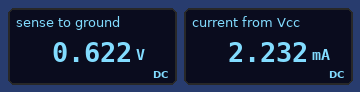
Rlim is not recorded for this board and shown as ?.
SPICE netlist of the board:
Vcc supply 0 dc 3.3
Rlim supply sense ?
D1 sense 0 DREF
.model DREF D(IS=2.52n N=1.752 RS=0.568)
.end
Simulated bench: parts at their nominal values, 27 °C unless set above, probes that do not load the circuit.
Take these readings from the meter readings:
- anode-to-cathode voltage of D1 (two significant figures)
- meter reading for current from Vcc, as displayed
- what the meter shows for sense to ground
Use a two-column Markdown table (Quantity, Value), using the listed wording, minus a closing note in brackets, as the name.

| Quantity | Value |
|---|---|
| anode-to-cathode voltage of D1 | 620 mV |
| meter reading for current from Vcc, as displayed | 2.232 mA |
| what the meter shows for sense to ground | 0.622 V |
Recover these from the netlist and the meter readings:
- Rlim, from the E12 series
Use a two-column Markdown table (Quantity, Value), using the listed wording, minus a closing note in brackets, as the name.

| Quantity | Value |
|---|---|
| Rlim, from the E12 series | 1.2 kΩ |
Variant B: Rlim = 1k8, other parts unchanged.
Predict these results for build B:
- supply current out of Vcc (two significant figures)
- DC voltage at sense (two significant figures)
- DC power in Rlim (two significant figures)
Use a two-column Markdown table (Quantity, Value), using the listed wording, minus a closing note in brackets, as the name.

| Quantity | Value |
|---|---|
| supply current out of Vcc | 1.5 mA |
| DC voltage at sense | 600 mV |
| DC power in Rlim | 4.0 mW |
